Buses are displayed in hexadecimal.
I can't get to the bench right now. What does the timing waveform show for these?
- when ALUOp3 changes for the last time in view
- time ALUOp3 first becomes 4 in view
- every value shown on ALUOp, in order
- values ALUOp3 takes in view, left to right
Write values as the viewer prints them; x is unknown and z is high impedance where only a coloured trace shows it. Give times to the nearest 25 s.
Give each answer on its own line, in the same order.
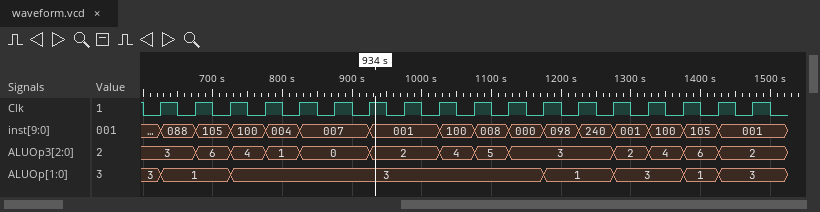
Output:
1425 s
725 s
3, 1, 3, 1, 3, 1, 3
3, 6, 4, 1, 0, 2, 4, 5, 3, 2, 4, 6, 2
